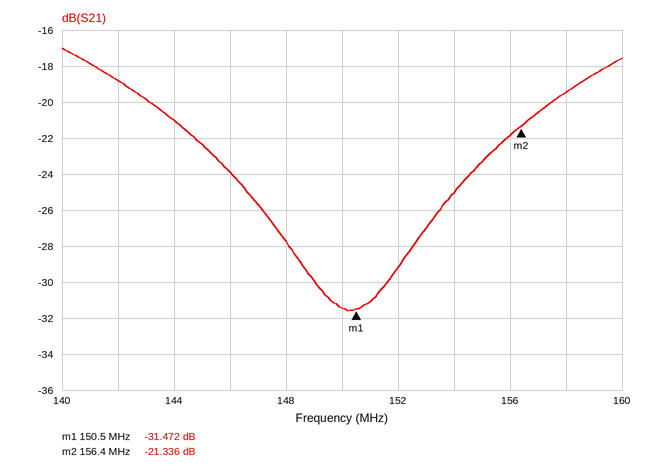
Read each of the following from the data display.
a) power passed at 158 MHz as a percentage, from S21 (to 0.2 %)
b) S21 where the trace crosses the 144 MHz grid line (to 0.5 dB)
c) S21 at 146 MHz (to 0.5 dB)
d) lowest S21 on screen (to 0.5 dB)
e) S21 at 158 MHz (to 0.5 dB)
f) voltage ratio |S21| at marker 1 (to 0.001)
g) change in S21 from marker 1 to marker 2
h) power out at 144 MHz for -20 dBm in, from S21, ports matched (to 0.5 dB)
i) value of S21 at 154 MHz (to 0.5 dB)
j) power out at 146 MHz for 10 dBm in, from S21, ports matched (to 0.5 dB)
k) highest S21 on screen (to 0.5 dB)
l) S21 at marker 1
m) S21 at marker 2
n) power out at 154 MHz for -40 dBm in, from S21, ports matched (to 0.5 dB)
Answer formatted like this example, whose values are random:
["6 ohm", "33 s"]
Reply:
["1.2 %", "-21.0 dB", "-24.0 dB", "-31.5 dB", "-19.5 dB", "0.027", "10.136 dB", "-41.0 dBm", "-25.0 dB", "-14.0 dBm", "-17.0 dB", "-31.472 dB", "-21.336 dB", "-65.0 dBm"]
